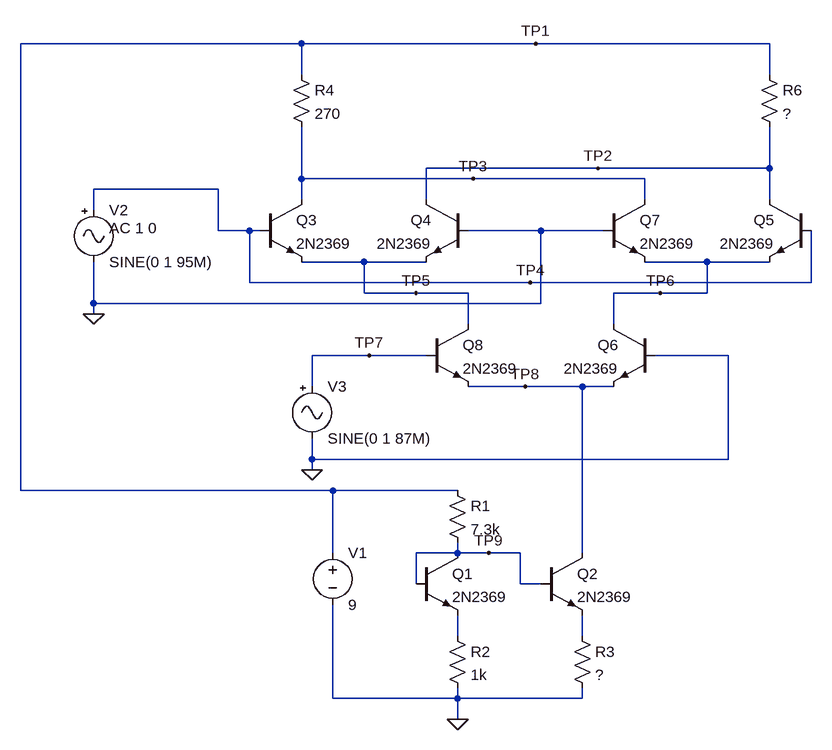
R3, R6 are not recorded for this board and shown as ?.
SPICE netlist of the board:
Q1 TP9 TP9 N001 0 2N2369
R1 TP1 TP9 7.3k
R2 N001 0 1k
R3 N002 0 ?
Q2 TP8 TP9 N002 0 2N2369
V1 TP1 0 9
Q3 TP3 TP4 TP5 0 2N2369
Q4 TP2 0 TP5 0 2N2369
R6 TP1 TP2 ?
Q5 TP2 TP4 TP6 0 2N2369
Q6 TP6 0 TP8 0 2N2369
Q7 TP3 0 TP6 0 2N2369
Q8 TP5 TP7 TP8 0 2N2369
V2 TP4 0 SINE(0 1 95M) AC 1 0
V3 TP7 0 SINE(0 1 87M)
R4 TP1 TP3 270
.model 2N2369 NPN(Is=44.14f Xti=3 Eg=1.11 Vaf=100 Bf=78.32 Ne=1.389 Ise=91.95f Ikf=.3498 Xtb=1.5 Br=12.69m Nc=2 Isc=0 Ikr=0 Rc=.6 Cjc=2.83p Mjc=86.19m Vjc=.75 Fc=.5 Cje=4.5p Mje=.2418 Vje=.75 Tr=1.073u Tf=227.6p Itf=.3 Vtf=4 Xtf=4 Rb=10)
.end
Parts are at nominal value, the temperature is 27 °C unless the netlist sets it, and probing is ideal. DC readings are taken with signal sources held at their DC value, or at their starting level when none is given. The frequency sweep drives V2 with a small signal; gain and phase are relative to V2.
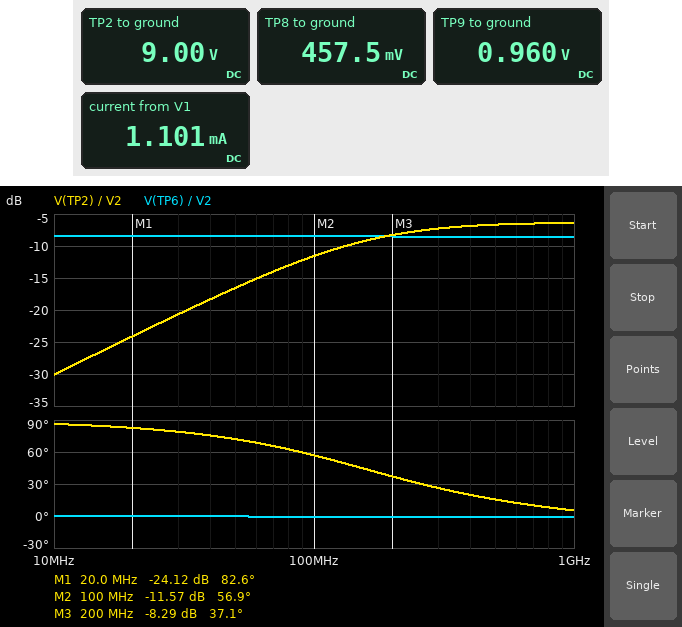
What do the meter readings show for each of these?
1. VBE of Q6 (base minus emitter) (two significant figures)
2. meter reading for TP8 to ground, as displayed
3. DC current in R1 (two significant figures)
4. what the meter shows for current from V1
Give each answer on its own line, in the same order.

-460 mV
457.5 mV
1.1 mA
1.101 mA
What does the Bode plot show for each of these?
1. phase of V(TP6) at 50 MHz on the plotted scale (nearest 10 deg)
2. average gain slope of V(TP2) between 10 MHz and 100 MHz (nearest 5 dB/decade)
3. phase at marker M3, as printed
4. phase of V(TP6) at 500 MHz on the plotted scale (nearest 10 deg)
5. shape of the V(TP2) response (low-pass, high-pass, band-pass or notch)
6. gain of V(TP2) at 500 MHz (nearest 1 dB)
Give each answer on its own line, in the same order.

0 deg
20 dB/decade
37.1 deg
0 deg
high-pass
-7 dB
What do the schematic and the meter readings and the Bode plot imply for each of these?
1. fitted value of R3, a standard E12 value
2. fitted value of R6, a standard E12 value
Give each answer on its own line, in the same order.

470 Ω
220 Ω
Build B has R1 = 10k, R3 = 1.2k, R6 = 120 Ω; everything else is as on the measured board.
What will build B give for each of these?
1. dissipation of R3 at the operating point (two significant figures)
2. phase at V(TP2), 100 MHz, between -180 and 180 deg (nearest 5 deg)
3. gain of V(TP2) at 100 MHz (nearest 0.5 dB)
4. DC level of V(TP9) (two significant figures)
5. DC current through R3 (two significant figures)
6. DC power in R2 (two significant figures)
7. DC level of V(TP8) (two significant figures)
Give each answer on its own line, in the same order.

160 µW
70 deg
-16.0 dB
1.0 V
360 µA
190 µW
550 mV
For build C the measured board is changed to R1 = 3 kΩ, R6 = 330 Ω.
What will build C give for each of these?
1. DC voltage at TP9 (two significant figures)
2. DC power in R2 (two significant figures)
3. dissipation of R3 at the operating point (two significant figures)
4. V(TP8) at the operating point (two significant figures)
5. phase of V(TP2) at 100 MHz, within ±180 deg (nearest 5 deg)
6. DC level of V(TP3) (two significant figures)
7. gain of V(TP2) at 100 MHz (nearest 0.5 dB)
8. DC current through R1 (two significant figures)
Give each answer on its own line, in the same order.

1.4 V
690 µW
1.3 mW
910 mV
45 deg
9.0 V
-9.5 dB
2.5 mA
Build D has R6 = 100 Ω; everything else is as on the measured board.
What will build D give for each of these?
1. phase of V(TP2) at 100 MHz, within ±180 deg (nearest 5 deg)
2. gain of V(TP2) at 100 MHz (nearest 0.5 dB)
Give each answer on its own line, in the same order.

75 deg
-17.5 dB
